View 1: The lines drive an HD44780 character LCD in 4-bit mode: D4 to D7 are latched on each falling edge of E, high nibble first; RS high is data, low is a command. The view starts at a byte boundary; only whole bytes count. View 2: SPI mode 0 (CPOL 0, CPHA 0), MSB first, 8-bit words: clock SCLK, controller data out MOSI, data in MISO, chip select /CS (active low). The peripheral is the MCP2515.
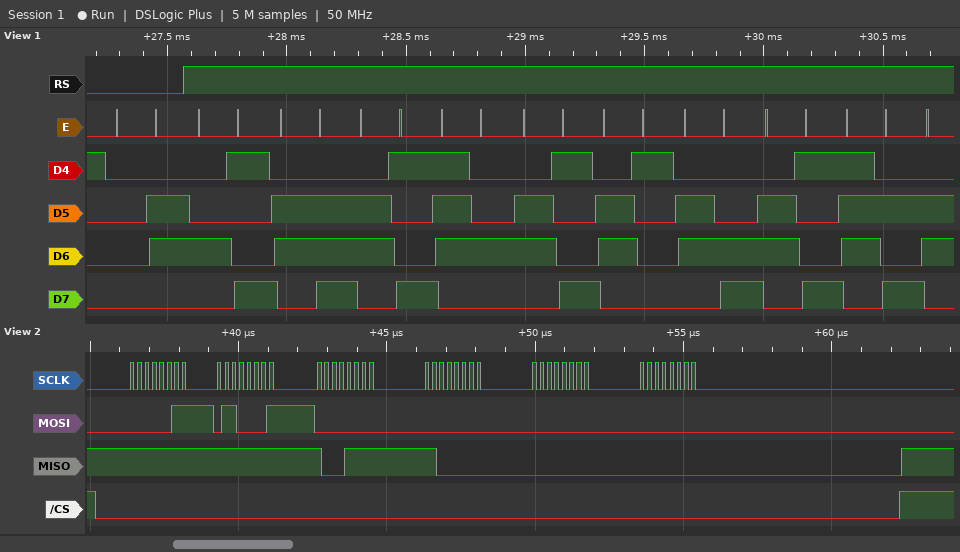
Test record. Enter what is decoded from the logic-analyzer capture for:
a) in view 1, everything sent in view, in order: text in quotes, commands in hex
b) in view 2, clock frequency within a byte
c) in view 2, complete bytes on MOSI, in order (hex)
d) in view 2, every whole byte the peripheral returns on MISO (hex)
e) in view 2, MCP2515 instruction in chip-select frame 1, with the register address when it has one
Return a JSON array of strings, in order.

["0x06 \"Initializ\"", "4 MHz", "0x03 0x61 0x00 0x00 0x00 0x00", "0xFF 0xFF 0x8F 0xC0 0x00 0x00", "READ 0x61"]
